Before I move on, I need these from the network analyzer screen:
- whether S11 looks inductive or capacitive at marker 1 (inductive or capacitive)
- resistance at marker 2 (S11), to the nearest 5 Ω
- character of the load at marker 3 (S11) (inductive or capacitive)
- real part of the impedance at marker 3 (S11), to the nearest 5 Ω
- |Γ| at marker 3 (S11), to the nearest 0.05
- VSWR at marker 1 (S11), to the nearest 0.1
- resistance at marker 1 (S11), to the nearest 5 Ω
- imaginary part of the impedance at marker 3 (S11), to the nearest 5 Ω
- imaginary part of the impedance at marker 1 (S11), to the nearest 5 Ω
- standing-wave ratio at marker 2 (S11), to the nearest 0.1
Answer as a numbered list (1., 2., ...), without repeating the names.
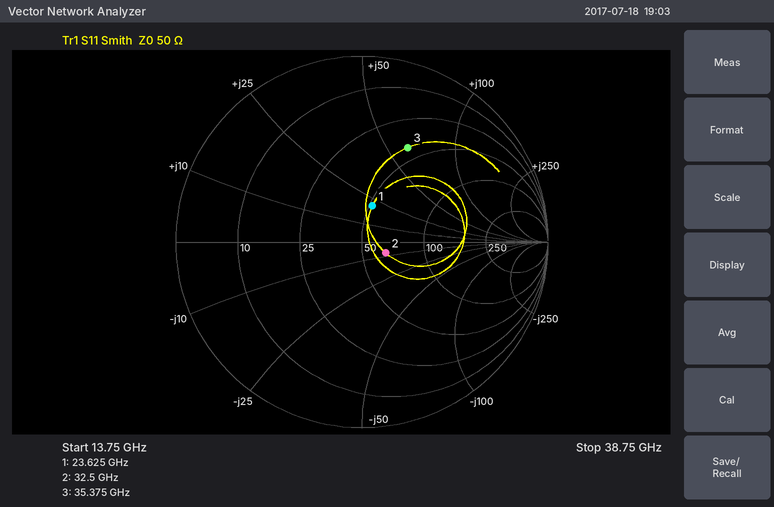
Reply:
1. inductive
2. 65 Ω
3. inductive
4. 40 Ω
5. 0.55
6. 1.5
7. 50 Ω
8. +60 Ω
9. +20 Ω
10. 1.3
